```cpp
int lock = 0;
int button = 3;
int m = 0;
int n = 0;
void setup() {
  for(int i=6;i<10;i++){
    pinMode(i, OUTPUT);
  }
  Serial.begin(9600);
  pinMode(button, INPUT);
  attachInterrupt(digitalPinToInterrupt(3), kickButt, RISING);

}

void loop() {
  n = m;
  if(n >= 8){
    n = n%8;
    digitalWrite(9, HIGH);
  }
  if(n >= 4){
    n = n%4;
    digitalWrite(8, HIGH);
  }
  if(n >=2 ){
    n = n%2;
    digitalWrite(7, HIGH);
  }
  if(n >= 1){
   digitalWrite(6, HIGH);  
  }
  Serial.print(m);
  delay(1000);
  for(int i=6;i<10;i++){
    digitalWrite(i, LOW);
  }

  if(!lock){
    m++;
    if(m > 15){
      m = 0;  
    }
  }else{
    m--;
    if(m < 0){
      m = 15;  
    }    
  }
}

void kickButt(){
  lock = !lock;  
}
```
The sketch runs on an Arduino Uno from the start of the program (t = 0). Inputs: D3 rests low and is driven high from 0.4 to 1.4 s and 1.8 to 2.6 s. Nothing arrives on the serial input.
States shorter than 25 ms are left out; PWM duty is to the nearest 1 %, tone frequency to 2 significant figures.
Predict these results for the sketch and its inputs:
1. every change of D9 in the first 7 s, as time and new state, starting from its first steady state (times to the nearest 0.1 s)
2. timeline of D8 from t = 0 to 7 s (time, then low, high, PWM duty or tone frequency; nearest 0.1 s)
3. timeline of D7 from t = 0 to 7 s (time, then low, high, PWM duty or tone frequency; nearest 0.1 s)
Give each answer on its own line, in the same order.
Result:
0 s low; 1 s high; 2 s low
0 s low; 1 s high; 2 s low; 6 s high
0 s low; 1 s high; 2 s low; 4 s high; 6 s low
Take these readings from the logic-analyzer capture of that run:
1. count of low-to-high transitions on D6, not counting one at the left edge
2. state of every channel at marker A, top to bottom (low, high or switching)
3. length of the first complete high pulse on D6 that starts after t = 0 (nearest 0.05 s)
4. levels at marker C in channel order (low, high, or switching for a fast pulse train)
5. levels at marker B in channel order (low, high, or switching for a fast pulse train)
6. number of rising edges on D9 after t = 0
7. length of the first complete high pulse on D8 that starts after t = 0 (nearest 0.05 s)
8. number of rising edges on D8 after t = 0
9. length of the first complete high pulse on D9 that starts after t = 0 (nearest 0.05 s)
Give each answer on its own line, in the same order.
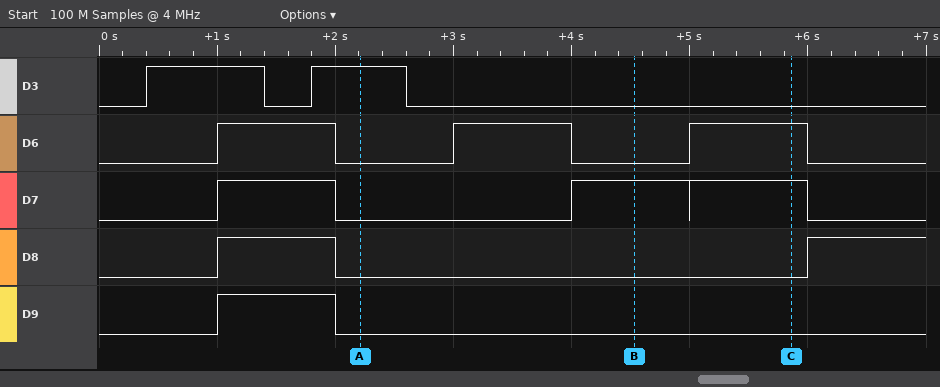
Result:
3
D3 high, D6 low, D7 low, D8 low, D9 low
1.00 s
D3 low, D6 high, D7 high, D8 low, D9 low
D3 low, D6 low, D7 high, D8 low, D9 low
1
1.00 s
2
1.00 s
